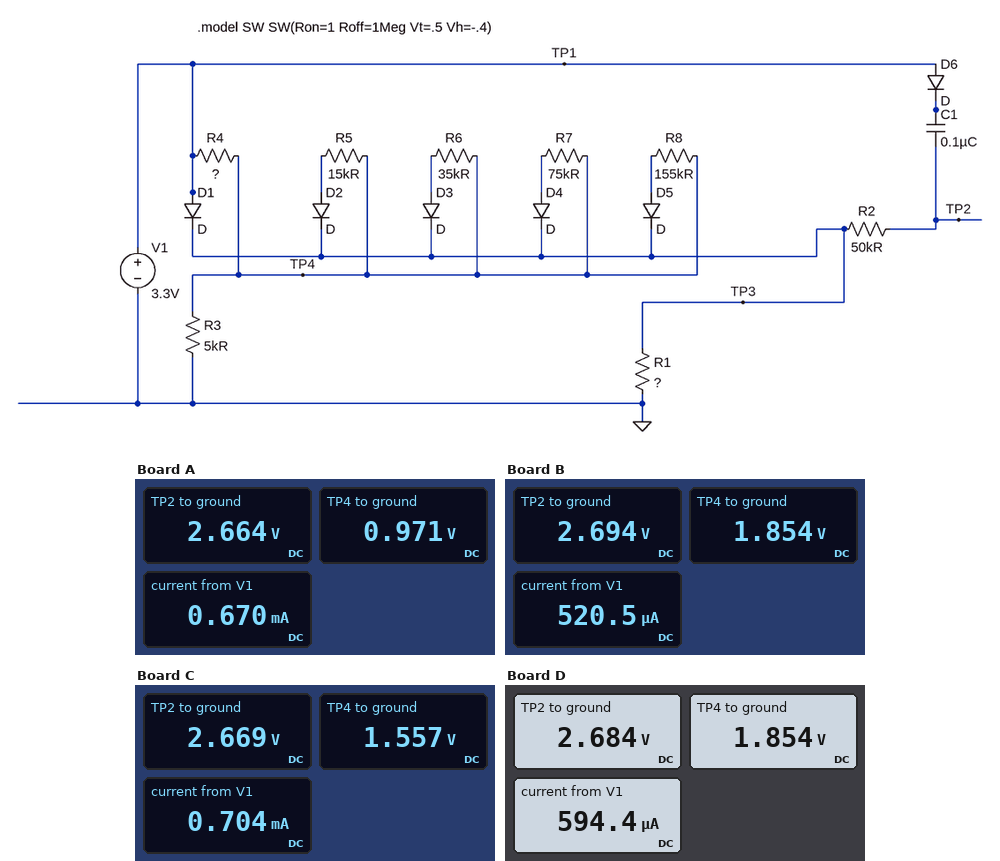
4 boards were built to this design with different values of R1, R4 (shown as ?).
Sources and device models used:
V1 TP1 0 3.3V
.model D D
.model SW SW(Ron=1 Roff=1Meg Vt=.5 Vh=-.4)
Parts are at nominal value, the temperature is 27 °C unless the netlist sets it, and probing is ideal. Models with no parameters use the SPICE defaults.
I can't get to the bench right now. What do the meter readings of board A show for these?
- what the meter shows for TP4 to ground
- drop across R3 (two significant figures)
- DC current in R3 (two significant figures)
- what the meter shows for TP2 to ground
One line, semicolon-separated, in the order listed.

0.971 V; 970 mV; 190 µA; 2.664 V
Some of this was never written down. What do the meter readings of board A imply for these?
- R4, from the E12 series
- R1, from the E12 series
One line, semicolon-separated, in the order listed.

12 kΩ; 5.6 kΩ
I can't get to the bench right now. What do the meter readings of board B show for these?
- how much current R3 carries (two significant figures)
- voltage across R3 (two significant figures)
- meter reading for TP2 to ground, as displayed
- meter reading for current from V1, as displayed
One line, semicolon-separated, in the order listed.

370 µA; 1.9 V; 2.694 V; 520.5 µA
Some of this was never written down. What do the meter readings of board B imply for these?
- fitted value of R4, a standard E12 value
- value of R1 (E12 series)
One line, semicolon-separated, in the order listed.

3.9 kΩ; 18 kΩ
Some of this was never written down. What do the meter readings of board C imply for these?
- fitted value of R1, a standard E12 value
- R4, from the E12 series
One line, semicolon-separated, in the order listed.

6.8 kΩ; 5.6 kΩ
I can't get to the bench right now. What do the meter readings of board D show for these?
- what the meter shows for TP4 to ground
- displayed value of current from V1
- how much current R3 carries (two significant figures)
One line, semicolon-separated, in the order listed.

1.854 V; 594.4 µA; 370 µA
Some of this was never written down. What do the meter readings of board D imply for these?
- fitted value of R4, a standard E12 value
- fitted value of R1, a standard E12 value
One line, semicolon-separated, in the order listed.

3.9 kΩ; 12 kΩ
